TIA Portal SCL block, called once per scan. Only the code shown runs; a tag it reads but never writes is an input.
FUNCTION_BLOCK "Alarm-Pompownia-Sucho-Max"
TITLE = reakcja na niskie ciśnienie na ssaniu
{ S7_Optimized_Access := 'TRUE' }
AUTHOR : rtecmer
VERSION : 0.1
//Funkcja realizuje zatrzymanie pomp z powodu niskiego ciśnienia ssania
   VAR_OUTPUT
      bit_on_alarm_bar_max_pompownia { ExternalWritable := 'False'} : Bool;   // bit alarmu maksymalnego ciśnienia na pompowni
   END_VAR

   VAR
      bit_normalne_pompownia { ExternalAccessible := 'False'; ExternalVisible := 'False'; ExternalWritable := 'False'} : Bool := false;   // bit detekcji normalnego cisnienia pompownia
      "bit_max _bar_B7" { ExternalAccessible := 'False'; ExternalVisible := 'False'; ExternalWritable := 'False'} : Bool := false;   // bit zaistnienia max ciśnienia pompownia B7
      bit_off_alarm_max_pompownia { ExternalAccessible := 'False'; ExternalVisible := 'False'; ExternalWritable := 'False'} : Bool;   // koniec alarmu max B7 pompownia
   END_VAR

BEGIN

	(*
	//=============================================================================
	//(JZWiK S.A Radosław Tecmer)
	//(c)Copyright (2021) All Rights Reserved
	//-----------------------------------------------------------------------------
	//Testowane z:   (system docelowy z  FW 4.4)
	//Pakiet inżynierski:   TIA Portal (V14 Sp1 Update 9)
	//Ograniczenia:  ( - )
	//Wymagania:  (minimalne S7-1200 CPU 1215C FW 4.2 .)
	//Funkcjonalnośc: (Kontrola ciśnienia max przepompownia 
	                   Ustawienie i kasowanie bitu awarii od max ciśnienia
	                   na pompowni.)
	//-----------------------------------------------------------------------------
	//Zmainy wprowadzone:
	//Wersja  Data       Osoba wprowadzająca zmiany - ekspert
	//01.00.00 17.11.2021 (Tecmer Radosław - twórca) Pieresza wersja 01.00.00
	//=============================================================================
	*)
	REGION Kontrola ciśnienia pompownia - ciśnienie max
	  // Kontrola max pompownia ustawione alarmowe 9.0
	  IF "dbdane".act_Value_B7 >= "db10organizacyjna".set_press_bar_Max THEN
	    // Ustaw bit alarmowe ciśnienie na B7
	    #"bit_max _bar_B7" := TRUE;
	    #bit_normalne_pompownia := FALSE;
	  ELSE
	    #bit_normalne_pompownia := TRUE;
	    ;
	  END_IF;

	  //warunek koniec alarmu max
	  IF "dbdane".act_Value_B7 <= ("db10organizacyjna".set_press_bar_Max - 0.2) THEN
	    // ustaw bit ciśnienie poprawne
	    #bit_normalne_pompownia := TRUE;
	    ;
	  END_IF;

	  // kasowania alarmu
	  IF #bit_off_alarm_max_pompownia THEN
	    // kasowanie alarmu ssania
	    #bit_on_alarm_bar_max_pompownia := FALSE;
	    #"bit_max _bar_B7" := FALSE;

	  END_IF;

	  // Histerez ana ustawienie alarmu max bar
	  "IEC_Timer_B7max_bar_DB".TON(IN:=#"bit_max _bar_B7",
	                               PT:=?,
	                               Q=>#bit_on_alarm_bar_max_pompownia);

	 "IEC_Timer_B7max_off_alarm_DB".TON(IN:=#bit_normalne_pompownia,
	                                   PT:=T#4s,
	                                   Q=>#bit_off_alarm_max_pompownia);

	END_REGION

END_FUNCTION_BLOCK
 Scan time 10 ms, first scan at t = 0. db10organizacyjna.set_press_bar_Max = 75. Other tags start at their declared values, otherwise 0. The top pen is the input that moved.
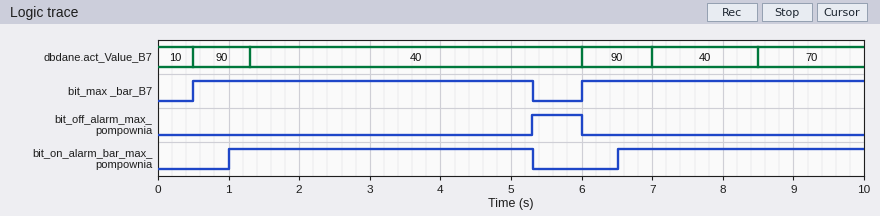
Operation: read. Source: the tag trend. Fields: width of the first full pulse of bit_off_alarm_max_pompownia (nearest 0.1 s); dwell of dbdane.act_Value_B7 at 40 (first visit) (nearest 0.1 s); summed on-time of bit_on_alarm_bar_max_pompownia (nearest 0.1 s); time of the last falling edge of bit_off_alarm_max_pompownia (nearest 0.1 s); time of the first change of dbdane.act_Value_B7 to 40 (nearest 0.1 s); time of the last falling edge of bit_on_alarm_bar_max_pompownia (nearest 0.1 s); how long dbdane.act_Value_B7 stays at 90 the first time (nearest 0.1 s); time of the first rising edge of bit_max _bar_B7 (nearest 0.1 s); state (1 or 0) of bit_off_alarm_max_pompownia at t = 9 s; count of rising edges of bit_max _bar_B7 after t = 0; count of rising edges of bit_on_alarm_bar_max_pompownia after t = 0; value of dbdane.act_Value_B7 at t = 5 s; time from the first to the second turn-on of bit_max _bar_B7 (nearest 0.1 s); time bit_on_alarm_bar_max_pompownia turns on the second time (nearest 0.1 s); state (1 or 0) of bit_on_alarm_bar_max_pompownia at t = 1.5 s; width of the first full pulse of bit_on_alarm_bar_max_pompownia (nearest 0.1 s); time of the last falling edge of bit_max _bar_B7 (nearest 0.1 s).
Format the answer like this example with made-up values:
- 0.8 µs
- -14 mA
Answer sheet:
- 0.7 s
- 4.7 s
- 7.8 s
- 6.0 s
- 1.3 s
- 5.3 s
- 0.8 s
- 0.5 s
- 0
- 2
- 2
- 40
- 5.5 s
- 6.5 s
- 1
- 4.3 s
- 5.3 s
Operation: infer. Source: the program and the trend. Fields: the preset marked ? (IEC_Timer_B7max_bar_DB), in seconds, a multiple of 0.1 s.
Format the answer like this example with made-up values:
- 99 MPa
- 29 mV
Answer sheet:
- 0.5 s
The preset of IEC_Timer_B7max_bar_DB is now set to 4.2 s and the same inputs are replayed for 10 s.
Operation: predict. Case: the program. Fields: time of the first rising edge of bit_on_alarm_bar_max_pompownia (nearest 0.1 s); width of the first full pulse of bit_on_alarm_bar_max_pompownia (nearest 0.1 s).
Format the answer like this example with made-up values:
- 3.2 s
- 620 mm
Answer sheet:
- 4.7 s
- 0.6 s
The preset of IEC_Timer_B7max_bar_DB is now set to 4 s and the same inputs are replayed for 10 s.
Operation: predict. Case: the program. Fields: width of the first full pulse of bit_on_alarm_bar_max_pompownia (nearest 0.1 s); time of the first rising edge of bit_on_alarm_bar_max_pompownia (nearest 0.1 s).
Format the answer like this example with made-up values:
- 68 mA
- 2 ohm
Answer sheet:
- 0.8 s
- 4.5 s
